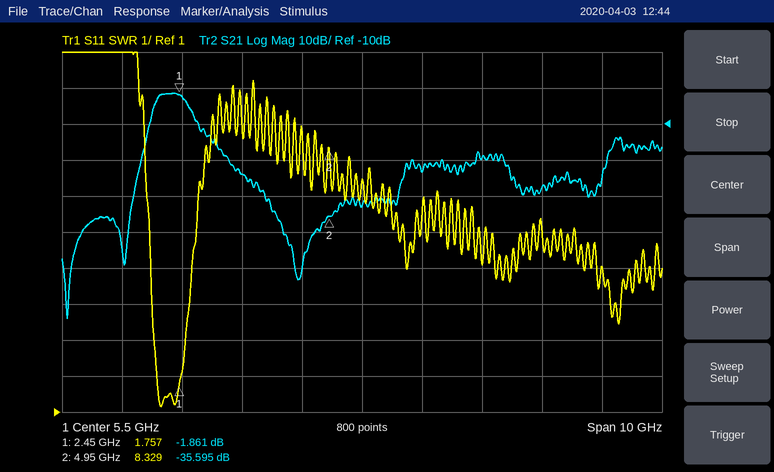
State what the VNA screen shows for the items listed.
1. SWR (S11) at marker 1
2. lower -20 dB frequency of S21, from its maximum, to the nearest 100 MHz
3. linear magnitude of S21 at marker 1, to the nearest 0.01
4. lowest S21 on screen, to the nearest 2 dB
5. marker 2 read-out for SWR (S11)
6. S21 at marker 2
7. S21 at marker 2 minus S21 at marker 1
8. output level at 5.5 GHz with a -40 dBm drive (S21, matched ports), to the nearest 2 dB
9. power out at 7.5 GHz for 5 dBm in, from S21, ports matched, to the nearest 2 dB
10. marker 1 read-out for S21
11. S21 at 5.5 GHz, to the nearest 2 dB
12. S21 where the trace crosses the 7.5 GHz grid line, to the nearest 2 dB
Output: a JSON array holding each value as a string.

["1.757", "1.8 GHz", "0.81", "-64 dB", "8.329", "-35.595 dB", "-33.734 dB", "-72 dBm", "-14 dBm", "-1.861 dB", "-32 dB", "-20 dB"]
